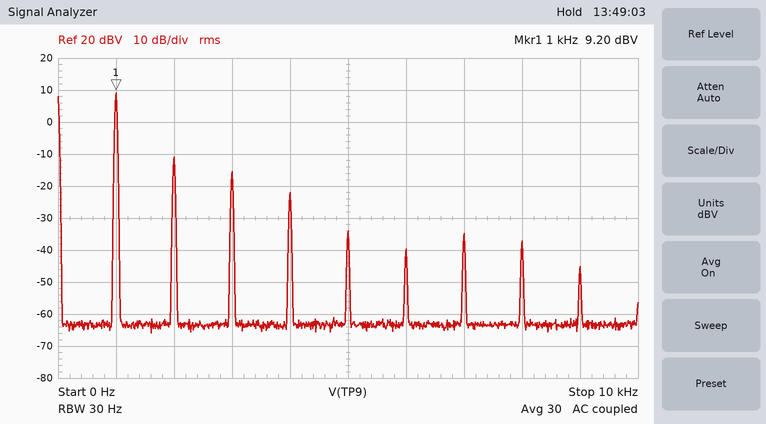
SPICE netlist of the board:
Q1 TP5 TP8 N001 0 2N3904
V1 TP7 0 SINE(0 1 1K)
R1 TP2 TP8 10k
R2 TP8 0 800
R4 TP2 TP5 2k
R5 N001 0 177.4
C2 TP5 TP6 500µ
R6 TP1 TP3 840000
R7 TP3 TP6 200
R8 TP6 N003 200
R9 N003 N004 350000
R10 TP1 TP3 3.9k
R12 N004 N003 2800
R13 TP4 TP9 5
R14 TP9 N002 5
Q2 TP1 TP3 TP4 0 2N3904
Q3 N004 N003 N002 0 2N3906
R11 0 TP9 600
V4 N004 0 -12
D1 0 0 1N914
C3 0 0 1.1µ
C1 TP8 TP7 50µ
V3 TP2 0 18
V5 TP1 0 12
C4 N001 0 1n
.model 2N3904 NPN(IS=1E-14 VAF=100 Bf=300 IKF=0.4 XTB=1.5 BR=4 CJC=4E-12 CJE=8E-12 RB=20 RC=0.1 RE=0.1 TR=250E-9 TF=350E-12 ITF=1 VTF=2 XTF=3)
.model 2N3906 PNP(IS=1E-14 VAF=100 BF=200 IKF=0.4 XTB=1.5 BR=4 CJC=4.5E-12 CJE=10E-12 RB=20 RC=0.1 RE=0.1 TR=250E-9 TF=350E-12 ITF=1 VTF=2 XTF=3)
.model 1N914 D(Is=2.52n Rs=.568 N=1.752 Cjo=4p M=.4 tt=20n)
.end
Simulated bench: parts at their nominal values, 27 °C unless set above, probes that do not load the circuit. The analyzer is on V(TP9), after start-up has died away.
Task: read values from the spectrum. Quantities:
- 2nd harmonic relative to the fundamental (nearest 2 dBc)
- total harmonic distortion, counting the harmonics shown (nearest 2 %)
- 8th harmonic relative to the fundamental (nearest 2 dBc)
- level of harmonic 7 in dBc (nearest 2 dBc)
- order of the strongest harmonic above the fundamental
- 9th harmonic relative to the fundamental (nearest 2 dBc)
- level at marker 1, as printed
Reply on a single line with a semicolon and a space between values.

-20 dBc; 12 %; -46 dBc; -44 dBc; 2; -54 dBc; 9.20 dBV
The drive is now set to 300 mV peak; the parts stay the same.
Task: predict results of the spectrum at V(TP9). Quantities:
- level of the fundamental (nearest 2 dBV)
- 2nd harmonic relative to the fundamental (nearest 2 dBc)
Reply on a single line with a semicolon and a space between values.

0 dBV; -50 dBc
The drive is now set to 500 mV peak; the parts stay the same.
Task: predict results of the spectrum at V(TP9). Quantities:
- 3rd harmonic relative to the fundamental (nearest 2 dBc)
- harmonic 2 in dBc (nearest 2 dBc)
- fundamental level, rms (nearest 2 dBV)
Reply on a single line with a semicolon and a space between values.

-52 dBc; -42 dBc; 4 dBV
